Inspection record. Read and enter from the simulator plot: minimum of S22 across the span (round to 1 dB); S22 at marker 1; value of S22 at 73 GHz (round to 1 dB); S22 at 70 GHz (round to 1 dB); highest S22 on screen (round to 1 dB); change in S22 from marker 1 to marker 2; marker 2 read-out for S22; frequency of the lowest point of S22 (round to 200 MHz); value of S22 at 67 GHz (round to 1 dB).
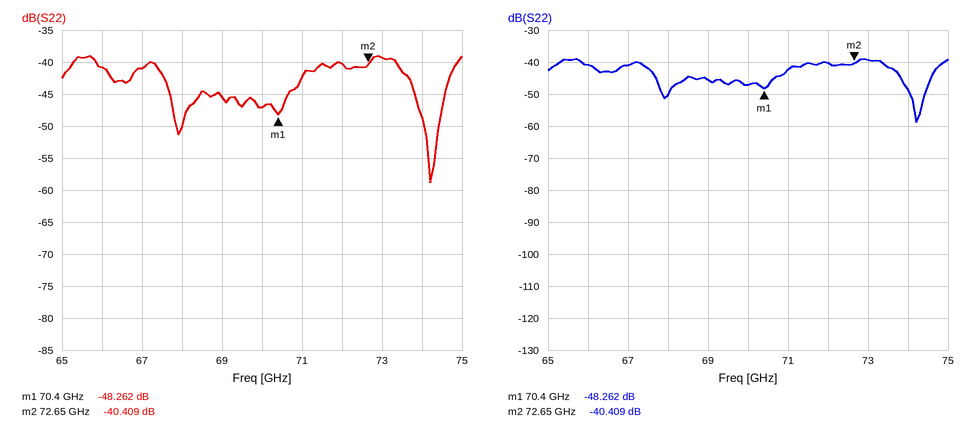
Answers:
-59 dB
-48.262 dB
-39 dB
-47 dB
-39 dB
7.853 dB
-40.409 dB
74.2 GHz
-41 dB
